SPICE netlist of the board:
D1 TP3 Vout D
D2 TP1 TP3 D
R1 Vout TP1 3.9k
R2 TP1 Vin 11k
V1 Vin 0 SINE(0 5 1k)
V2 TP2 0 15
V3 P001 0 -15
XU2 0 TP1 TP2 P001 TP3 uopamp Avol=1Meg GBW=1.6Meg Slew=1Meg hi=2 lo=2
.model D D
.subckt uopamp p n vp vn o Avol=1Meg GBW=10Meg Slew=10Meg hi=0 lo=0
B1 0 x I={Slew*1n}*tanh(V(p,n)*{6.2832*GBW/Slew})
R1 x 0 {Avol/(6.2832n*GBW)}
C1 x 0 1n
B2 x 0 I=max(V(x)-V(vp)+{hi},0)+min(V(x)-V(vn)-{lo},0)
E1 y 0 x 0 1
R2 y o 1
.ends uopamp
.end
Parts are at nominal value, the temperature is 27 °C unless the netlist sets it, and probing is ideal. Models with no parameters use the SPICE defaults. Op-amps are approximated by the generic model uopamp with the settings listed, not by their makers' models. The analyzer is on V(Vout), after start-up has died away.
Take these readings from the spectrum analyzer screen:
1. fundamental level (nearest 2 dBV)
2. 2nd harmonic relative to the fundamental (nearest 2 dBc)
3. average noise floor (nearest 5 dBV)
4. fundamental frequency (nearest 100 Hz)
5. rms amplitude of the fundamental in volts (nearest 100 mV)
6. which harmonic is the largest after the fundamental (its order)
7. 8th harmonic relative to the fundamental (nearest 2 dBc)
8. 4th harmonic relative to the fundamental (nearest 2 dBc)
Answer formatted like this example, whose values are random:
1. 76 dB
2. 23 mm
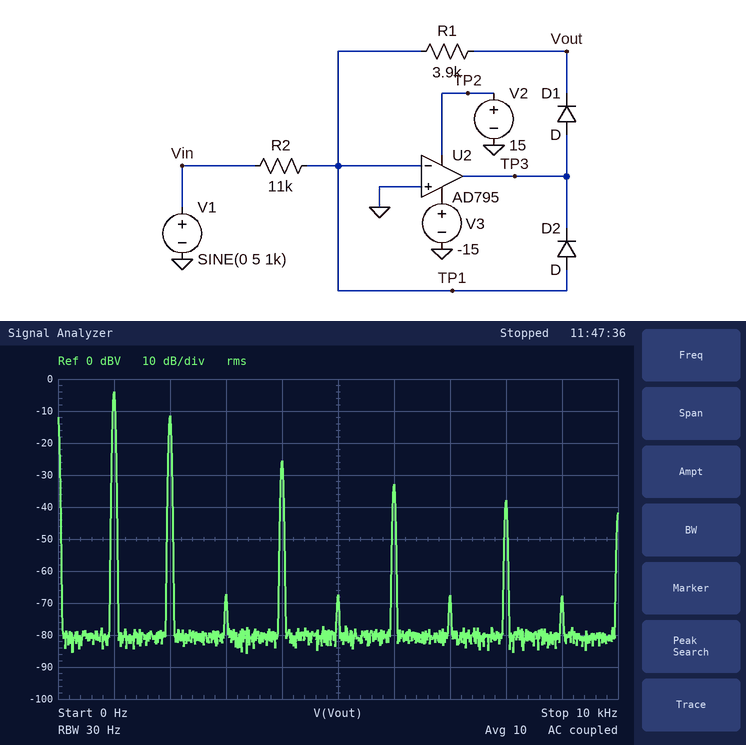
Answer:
1. -4 dBV
2. -8 dBc
3. -80 dBV
4. 1.0 kHz
5. 600 mV
6. 2
7. -34 dBc
8. -22 dBc
